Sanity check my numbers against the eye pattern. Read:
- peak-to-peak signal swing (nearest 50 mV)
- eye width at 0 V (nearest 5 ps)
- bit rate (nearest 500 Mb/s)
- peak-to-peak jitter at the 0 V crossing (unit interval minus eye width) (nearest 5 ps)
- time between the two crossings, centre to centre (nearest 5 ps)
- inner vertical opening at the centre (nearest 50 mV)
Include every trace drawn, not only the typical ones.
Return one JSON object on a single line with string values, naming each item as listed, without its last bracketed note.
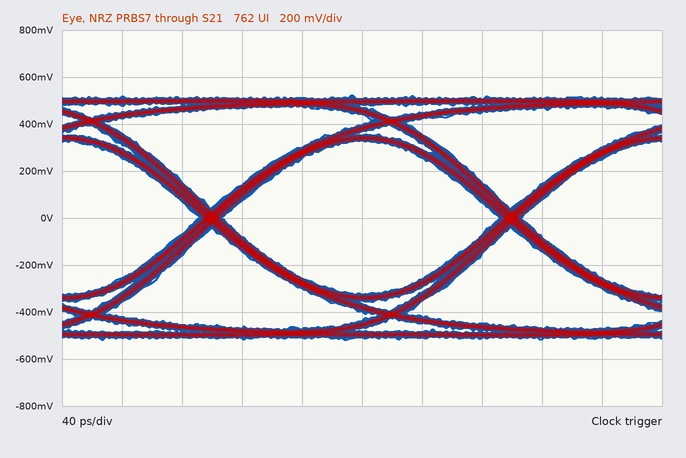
{"peak-to-peak signal swing": "1.05 V", "eye width at 0 V": "185 ps", "bit rate": "5.0 Gb/s", "peak-to-peak jitter at the 0 V crossing (unit interval minus eye width)": "15 ps", "time between the two crossings, centre to centre": "200 ps", "inner vertical opening at the centre": "650 mV"}
